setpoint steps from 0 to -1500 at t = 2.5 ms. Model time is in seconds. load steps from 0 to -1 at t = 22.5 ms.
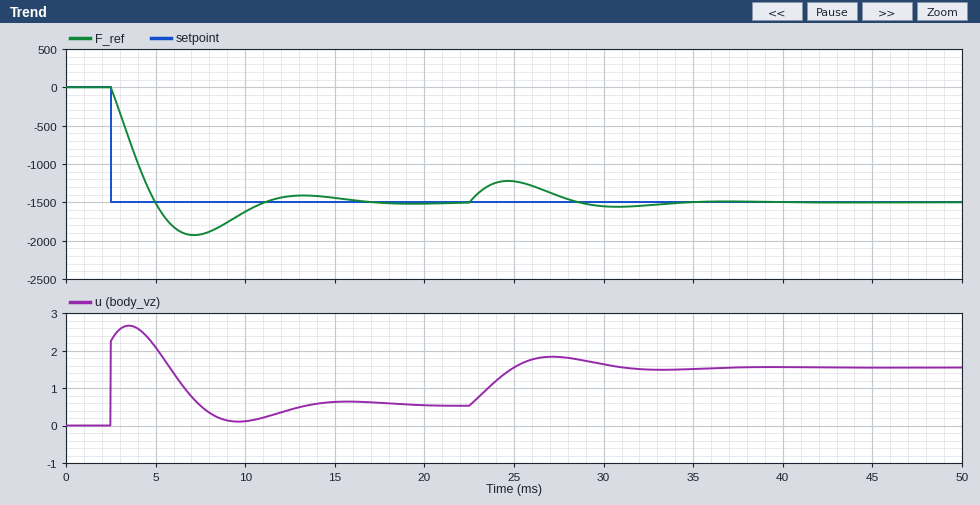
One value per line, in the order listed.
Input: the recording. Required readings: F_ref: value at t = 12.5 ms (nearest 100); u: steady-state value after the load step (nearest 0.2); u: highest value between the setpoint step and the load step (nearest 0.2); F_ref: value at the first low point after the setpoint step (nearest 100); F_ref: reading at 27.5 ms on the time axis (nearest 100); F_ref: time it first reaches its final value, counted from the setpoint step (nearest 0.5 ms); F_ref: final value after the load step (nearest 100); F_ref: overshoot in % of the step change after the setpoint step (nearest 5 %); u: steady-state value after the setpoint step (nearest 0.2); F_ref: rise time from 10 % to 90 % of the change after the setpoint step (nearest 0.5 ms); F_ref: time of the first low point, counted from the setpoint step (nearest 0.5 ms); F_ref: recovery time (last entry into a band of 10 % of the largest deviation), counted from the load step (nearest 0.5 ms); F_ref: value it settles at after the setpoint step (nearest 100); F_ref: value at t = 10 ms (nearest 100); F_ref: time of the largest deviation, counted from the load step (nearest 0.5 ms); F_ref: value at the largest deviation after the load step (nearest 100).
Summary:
-1400
1.6
2.6
-1900
-1400
2.5 ms
-1500
30 %
0.6
2.0 ms
4.5 ms
10.5 ms
-1500
-1600
2.0 ms
-1200
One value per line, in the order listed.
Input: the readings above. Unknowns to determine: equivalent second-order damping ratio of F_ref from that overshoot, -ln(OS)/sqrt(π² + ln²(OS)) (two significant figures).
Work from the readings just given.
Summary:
0.36
